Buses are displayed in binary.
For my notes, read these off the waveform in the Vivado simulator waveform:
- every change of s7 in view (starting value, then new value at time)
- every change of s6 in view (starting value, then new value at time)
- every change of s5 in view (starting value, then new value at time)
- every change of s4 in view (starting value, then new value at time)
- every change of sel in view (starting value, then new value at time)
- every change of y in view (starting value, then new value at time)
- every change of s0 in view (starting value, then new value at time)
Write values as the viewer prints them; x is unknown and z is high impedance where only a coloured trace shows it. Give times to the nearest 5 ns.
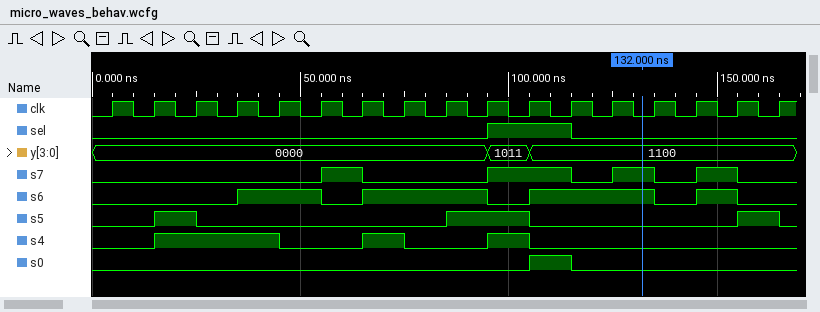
0, 1 at 55 ns, 0 at 65 ns, 1 at 95 ns, 0 at 115 ns, 1 at 125 ns, 0 at 135 ns, 1 at 145 ns, 0 at 155 ns
0, 1 at 35 ns, 0 at 55 ns, 1 at 65 ns, 0 at 95 ns, 1 at 105 ns, 0 at 135 ns, 1 at 145 ns, 0 at 155 ns
0, 1 at 15 ns, 0 at 25 ns, 1 at 85 ns, 0 at 105 ns, 1 at 155 ns, 0 at 165 ns
0, 1 at 15 ns, 0 at 45 ns, 1 at 65 ns, 0 at 75 ns, 1 at 95 ns, 0 at 105 ns
0, 1 at 95 ns, 0 at 115 ns
0000, 1011 at 95 ns, 1100 at 105 ns
0, 1 at 105 ns, 0 at 115 ns
